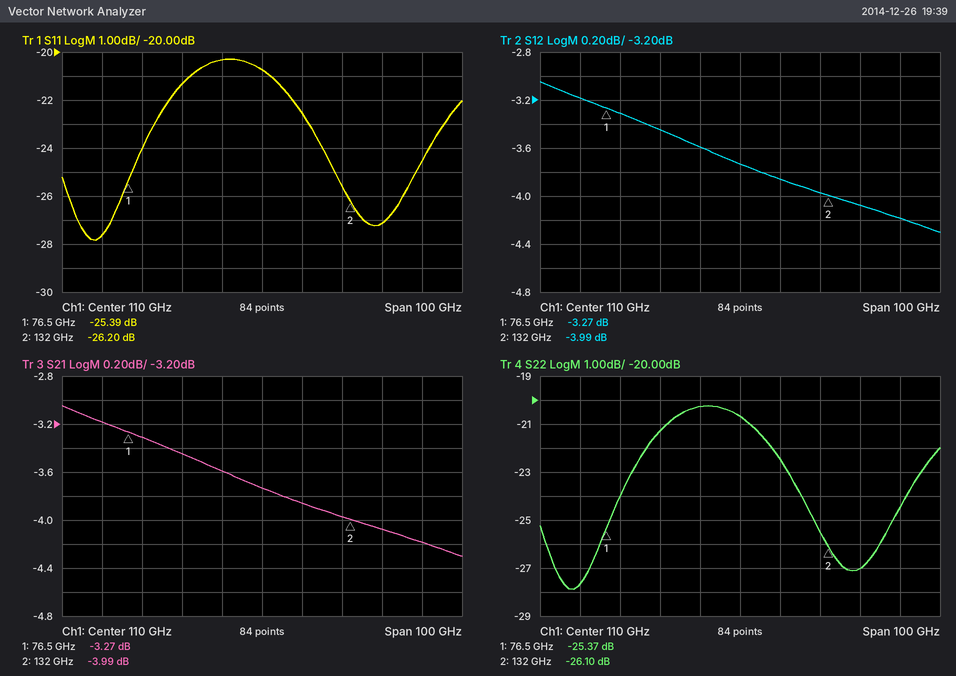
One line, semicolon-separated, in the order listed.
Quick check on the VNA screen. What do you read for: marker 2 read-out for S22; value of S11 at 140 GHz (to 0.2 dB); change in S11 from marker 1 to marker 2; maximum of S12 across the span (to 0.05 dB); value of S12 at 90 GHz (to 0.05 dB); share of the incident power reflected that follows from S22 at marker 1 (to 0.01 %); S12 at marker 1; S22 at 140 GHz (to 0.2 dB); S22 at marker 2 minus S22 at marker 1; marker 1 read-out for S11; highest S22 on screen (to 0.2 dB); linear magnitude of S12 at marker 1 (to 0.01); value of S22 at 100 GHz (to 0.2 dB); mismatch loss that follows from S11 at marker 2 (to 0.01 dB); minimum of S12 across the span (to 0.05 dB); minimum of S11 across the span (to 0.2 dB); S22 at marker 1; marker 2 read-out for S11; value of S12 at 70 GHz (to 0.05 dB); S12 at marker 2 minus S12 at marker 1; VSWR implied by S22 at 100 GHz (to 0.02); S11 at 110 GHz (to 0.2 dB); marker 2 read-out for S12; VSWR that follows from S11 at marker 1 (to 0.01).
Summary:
-26.10 dB; -27.2 dB; -0.81 dB; -3.05 dB; -3.45 dB; 0.29 %; -3.27 dB; -27.0 dB; -0.73 dB; -25.39 dB; -20.2 dB; 0.69; -20.2 dB; 0.01 dB; -4.30 dB; -27.8 dB; -25.37 dB; -26.20 dB; -3.20 dB; -0.72 dB; 1.22; -20.8 dB; -3.99 dB; 1.11
